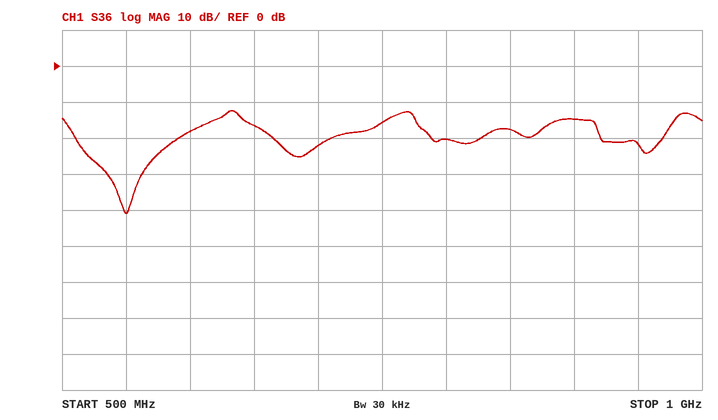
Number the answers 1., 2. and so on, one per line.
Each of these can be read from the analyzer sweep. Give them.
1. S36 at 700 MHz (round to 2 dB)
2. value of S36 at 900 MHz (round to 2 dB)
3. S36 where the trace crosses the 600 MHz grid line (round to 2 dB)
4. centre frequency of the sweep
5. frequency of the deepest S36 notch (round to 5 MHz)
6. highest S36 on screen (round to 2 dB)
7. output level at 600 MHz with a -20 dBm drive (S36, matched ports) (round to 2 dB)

1. -22 dB
2. -14 dB
3. -18 dB
4. 750 MHz
5. 550 MHz
6. -12 dB
7. -38 dBm
